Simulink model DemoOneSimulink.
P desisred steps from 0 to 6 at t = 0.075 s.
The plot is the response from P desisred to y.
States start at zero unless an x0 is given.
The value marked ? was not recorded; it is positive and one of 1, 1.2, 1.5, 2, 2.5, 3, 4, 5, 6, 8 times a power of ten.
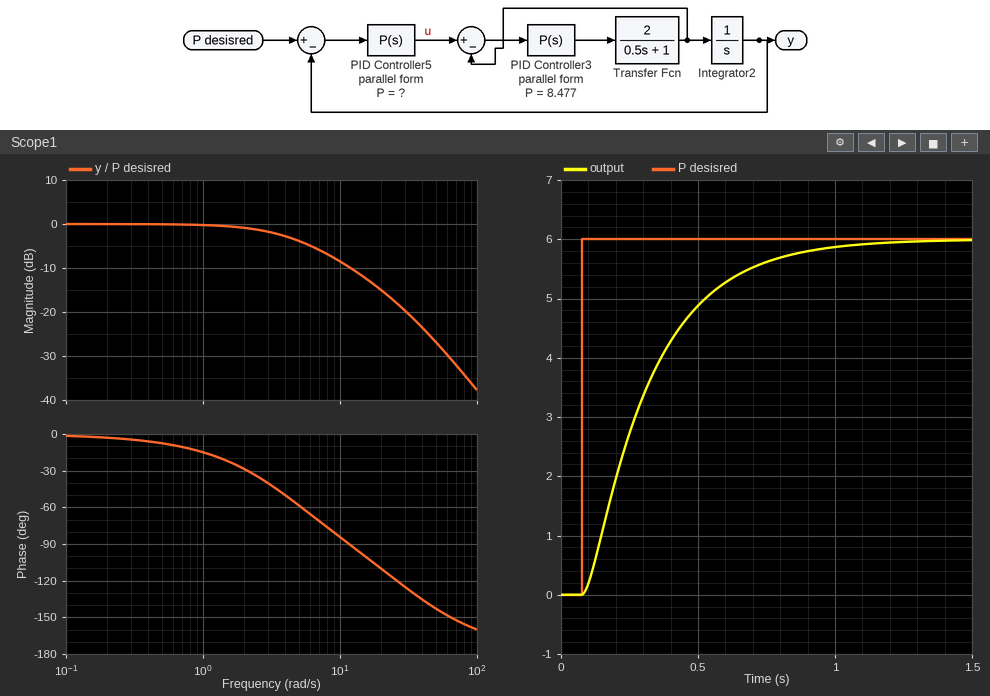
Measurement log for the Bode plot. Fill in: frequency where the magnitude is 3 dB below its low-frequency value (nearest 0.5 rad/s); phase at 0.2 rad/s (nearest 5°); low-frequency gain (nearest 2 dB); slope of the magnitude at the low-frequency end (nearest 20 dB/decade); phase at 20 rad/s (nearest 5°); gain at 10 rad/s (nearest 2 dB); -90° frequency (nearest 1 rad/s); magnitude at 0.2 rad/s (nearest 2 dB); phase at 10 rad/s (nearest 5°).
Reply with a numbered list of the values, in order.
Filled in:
1. 4.0 rad/s
2. -5°
3. 0 dB
4. 0 dB/decade
5. -110°
6. -8 dB
7. 12 rad/s
8. 0 dB
9. -85°
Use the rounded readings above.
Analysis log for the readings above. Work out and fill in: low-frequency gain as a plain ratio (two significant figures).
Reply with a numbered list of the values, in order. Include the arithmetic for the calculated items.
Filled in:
1. 10^(0 / 20) = 1.0
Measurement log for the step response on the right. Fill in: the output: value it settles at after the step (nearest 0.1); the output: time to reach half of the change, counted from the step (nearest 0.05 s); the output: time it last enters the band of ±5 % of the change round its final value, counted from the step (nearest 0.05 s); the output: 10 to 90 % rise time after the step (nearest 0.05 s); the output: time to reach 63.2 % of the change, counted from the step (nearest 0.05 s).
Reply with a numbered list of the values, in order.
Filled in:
1. 6.0
2. 0.20 s
3. 0.75 s
4. 0.50 s
5. 0.25 s
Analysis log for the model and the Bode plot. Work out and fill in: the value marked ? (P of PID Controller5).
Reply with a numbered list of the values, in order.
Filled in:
1. 4
